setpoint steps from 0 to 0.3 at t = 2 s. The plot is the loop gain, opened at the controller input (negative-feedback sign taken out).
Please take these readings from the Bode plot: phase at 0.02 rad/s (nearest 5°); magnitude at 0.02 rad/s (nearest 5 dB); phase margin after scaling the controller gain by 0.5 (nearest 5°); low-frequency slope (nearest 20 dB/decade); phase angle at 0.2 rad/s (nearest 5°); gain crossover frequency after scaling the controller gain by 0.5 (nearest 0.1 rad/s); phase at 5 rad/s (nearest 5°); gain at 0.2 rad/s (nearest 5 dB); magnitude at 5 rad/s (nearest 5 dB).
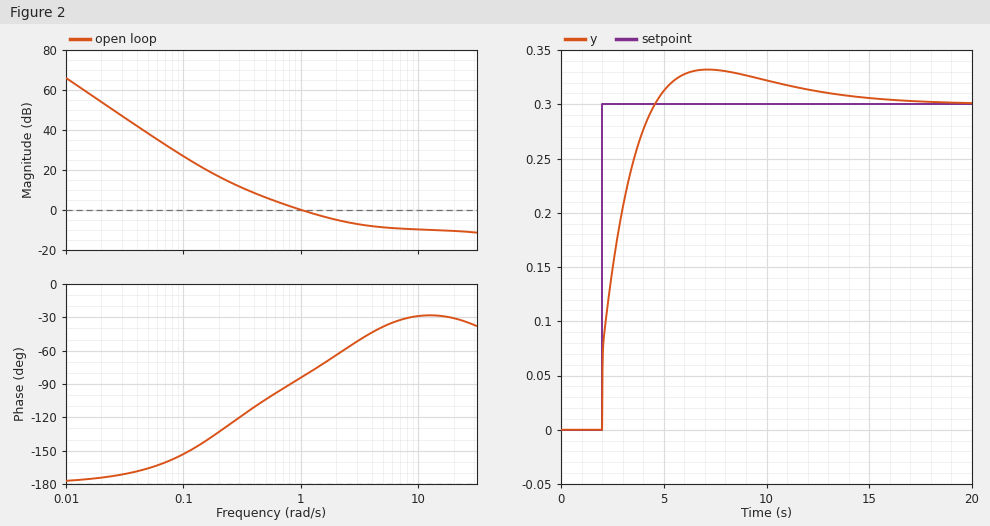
-175°
55 dB
75°
-40 dB/decade
-135°
0.5 rad/s
-40°
15 dB
-10 dB
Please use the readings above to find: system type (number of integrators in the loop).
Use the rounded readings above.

2
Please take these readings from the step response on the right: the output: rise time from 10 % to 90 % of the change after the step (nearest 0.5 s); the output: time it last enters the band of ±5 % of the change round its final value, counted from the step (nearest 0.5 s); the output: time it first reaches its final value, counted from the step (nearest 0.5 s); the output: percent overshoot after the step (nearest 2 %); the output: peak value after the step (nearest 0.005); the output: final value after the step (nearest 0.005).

2.0 s
9.5 s
2.5 s
10 %
0.330
0.300
